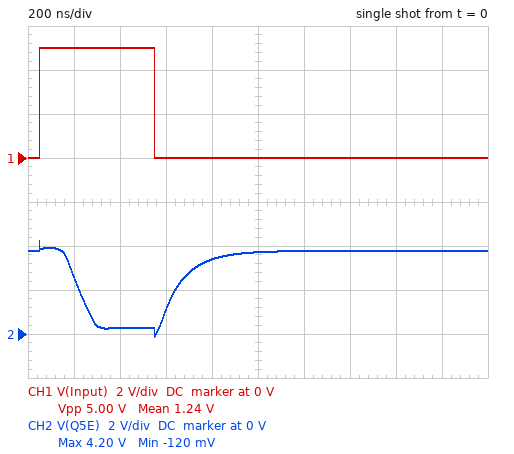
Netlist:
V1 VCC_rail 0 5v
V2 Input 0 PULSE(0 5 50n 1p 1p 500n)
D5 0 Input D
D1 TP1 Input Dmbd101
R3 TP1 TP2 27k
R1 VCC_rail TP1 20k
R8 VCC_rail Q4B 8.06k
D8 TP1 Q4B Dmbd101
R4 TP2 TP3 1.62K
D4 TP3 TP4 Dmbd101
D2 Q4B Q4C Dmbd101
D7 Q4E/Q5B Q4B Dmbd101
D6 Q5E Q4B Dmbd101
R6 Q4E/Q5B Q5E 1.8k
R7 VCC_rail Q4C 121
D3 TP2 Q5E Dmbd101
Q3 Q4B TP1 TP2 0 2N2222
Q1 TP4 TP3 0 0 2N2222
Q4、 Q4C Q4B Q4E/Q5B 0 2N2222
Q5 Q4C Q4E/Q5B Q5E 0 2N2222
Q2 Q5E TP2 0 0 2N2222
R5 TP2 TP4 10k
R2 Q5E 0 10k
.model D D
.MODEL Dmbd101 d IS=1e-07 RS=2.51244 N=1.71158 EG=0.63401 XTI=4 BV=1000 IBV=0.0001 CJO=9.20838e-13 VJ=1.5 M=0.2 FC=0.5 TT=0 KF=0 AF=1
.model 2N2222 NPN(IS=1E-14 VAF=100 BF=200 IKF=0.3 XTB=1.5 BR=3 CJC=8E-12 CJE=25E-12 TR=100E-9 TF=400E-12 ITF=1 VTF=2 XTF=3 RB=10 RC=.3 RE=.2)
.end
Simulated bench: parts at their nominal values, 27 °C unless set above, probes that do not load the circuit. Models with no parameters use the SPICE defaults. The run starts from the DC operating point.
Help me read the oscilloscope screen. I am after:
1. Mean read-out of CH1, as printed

1.24 V
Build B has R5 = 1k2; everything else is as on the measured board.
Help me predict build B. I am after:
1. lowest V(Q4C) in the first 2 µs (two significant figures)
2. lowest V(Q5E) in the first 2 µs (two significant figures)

3.6 V
-110 mV
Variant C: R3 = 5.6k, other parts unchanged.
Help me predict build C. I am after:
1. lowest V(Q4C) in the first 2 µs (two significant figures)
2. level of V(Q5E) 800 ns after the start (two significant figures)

1.5 V
3.5 V
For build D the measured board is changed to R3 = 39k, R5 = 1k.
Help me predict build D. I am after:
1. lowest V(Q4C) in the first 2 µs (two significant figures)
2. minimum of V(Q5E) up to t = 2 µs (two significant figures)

3.8 V
-110 mV
